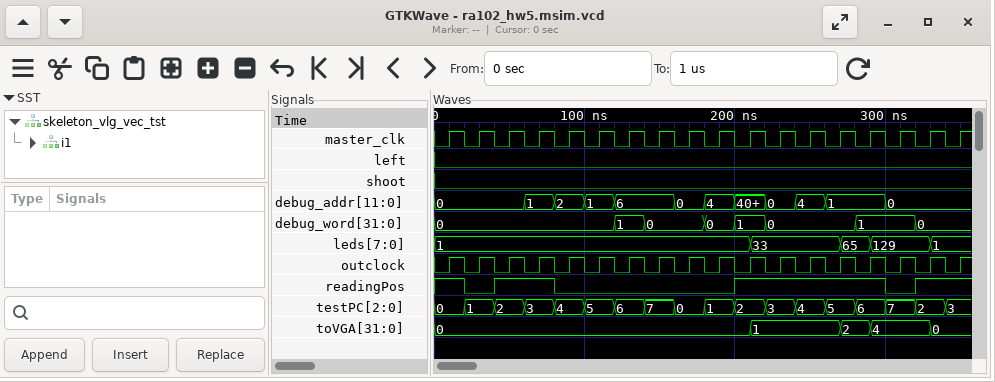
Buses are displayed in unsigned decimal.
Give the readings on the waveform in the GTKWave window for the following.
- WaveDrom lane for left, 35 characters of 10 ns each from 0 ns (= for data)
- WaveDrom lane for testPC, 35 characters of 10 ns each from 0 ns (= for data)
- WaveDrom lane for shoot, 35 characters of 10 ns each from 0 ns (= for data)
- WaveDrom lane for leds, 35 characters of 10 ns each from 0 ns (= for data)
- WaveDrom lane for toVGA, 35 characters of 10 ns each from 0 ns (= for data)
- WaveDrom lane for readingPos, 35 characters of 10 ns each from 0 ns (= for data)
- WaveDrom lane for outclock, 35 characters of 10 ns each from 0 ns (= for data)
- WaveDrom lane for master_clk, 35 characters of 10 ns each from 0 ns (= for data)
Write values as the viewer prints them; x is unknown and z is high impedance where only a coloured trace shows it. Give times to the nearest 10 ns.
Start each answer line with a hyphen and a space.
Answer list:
- {name: 'left', wave: '0..................................'}
- {name: 'testPC', wave: '=.=.=.=.=.=.=.=.=.=.=.=.=.=.=.=.=.=', data: '0 1 2 3 4 5 6 7 0 1 2 3 4 5 6 7 2 3'}
- {name: 'shoot', wave: '0..................................'}
- {name: 'leds', wave: '=....................=.....=.=...=.', data: '1 33 65 129 1'}
- {name: 'toVGA', wave: '=....................=.....=.=...=.', data: '0 1 2 4 0'}
- {name: 'readingPos', wave: '1.0.1...0...........1.........0.1..'}
- {name: 'outclock', wave: '01010101010101010101010101010101010'}
- {name: 'master_clk', wave: '01010101010101010101010101010101010'}
